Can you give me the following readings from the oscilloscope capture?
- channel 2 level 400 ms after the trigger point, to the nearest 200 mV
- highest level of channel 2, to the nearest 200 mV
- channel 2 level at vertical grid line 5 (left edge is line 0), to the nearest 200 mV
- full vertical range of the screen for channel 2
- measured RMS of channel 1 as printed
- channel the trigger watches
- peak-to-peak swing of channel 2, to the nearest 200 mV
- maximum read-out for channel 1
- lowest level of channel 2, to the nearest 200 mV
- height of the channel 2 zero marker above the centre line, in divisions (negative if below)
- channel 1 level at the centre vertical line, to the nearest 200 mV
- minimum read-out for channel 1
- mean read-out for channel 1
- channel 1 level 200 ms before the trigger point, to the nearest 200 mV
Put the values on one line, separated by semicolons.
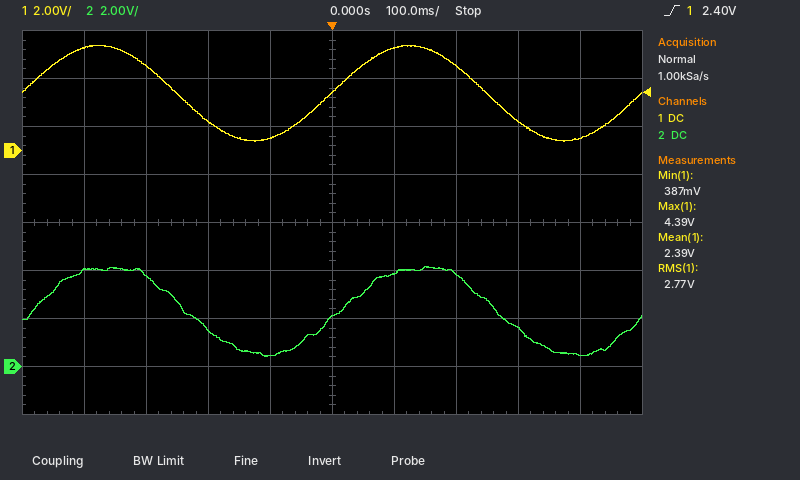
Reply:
400 mV; 4.2 V; 2.0 V; 16 V; 2.77 V; channel 1; 3.8 V; 4.39 V; 400 mV; -3.0 div; 2.4 V; 387 mV; 2.39 V; 1.2 V
